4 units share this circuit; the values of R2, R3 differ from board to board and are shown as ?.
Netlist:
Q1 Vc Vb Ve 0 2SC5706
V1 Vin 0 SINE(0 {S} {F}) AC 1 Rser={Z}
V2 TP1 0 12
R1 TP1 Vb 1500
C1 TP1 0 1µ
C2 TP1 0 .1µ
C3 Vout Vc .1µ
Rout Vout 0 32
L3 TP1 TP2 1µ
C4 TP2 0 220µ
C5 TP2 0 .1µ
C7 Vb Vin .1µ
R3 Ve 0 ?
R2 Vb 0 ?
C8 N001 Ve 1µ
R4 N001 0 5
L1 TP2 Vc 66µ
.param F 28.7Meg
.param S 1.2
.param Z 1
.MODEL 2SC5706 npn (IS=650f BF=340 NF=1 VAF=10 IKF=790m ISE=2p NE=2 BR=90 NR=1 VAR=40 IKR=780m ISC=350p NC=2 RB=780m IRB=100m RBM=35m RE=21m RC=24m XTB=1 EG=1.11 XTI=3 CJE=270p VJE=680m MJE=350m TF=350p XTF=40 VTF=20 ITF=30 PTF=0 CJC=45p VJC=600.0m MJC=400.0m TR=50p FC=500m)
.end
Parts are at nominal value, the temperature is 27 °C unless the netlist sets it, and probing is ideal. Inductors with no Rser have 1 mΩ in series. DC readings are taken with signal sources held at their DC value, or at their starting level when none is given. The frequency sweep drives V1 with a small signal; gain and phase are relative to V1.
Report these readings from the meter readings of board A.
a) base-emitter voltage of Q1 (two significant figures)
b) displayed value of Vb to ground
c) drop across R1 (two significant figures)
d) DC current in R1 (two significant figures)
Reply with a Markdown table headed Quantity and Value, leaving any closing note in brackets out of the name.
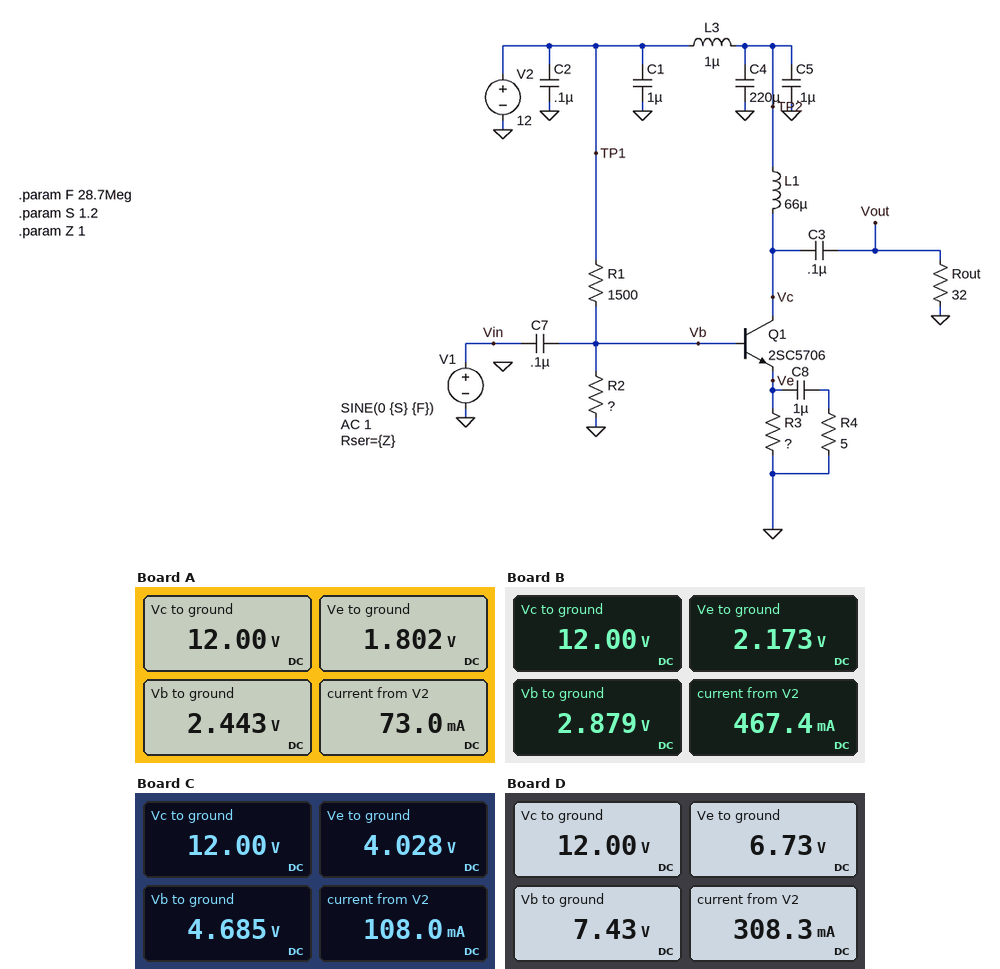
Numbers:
| Quantity | Value |
|---|---|
| base-emitter voltage of Q1 | 640 mV |
| displayed value of Vb to ground | 2.443 V |
| drop across R1 | 9.6 V |
| DC current in R1 | 6.4 mA |
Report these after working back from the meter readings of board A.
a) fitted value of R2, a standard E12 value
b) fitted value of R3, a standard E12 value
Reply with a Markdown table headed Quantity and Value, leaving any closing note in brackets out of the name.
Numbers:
| Quantity | Value |
|---|---|
| fitted value of R2, a standard E12 value | 390 Ω |
| fitted value of R3, a standard E12 value | 27 Ω |
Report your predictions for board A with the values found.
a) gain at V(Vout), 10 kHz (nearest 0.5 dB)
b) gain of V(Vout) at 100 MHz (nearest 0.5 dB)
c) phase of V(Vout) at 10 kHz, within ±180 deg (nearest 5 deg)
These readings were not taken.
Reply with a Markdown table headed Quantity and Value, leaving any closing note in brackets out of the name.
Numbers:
| Quantity | Value |
|---|---|
| gain at V(Vout), 10 kHz | -24.0 dB |
| gain of V(Vout) at 100 MHz | 15.0 dB |
| phase of V(Vout) at 10 kHz, within ±180 deg | 60 deg |
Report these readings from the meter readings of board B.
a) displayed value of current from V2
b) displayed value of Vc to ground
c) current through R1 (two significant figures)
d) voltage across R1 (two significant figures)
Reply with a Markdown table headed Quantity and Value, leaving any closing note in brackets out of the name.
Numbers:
| Quantity | Value |
|---|---|
| displayed value of current from V2 | 467.4 mA |
| displayed value of Vc to ground | 12.00 V |
| current through R1 | 6.1 mA |
| voltage across R1 | 9.1 V |
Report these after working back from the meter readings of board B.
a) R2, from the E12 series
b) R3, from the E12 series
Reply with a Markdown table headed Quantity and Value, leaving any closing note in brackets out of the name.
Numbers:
| Quantity | Value |
|---|---|
| R2, from the E12 series | 560 Ω |
| R3, from the E12 series | 4.7 Ω |
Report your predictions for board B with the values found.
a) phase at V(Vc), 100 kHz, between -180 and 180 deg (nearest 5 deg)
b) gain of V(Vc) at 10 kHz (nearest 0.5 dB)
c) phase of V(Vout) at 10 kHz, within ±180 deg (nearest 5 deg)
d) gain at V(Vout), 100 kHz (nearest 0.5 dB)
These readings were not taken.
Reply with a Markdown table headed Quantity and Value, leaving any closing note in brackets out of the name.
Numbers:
| Quantity | Value |
|---|---|
| phase at V(Vc), 100 kHz, between -180 and 180 deg | -145 deg |
| gain of V(Vc) at 10 kHz | -0.5 dB |
| phase of V(Vout) at 10 kHz, within ±180 deg | 25 deg |
| gain at V(Vout), 100 kHz | 21.5 dB |
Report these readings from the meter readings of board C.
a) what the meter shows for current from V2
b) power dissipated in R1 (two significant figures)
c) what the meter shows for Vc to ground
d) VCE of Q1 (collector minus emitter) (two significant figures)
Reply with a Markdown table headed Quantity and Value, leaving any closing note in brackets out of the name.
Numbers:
| Quantity | Value |
|---|---|
| what the meter shows for current from V2 | 108.0 mA |
| power dissipated in R1 | 36 mW |
| what the meter shows for Vc to ground | 12.00 V |
| VCE of Q1 (collector minus emitter) | 8.0 V |
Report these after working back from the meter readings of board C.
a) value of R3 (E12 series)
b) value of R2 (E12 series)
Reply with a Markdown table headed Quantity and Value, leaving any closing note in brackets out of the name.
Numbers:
| Quantity | Value |
|---|---|
| value of R3 | 39 Ω |
| value of R2 | 1 kΩ |
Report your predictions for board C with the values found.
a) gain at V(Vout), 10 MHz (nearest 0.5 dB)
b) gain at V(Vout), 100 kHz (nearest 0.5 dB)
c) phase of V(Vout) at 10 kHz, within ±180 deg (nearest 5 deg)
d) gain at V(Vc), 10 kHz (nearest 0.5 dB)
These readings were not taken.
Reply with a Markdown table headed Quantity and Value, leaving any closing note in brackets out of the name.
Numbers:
| Quantity | Value |
|---|---|
| gain at V(Vout), 10 MHz | 16.5 dB |
| gain at V(Vout), 100 kHz | 16.0 dB |
| phase of V(Vout) at 10 kHz, within ±180 deg | 55 deg |
| gain at V(Vc), 10 kHz | -10.0 dB |
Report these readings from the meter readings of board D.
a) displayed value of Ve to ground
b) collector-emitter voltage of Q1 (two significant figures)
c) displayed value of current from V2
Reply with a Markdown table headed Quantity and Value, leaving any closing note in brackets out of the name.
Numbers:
| Quantity | Value |
|---|---|
| displayed value of Ve to ground | 6.73 V |
| collector-emitter voltage of Q1 | 5.3 V |
| displayed value of current from V2 | 308.3 mA |
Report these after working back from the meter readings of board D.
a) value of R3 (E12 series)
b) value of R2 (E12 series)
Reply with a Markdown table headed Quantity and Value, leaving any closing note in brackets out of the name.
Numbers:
| Quantity | Value |
|---|---|
| value of R3 | 22 Ω |
| value of R2 | 3.3 kΩ |
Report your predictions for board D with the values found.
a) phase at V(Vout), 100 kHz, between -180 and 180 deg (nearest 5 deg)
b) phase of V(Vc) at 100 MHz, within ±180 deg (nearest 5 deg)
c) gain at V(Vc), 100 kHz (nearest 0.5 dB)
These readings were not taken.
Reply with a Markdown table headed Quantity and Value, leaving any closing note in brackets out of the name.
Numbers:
| Quantity | Value |
|---|---|
| phase at V(Vout), 100 kHz, between -180 and 180 deg | -115 deg |
| phase of V(Vc) at 100 MHz, within ±180 deg | 130 deg |
| gain at V(Vc), 100 kHz | 18.0 dB |
